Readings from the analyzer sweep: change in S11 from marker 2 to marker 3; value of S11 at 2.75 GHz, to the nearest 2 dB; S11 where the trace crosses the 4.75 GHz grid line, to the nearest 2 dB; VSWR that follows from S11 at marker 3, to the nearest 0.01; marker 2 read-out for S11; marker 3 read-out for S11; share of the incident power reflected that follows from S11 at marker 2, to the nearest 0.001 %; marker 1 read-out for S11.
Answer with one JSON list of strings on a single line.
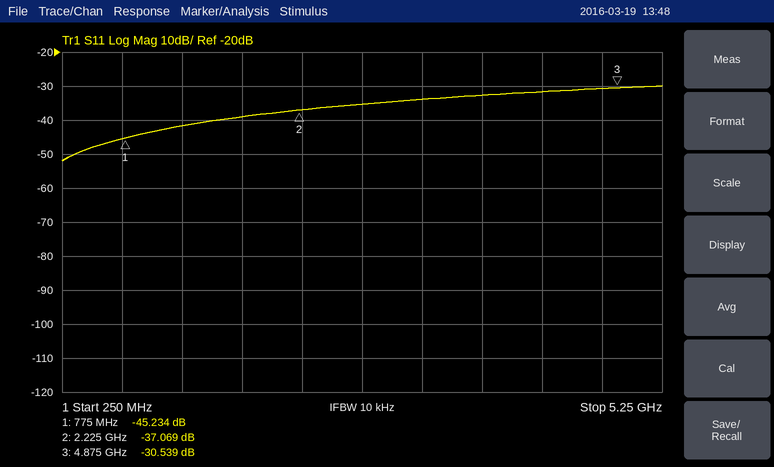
["6.530 dB", "-36 dB", "-30 dB", "1.06", "-37.069 dB", "-30.539 dB", "0.020 %", "-45.234 dB"]
